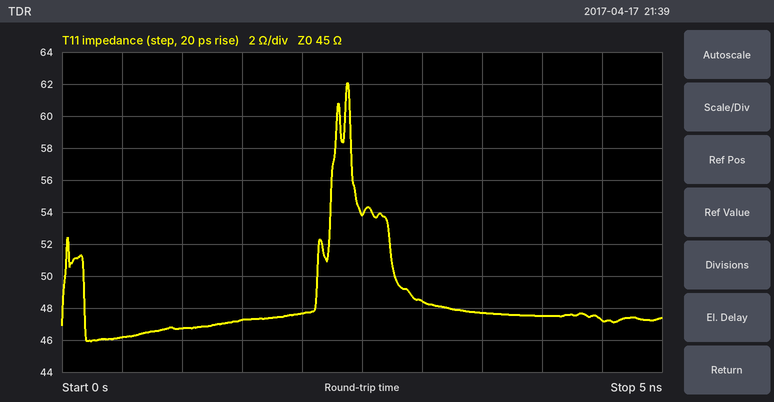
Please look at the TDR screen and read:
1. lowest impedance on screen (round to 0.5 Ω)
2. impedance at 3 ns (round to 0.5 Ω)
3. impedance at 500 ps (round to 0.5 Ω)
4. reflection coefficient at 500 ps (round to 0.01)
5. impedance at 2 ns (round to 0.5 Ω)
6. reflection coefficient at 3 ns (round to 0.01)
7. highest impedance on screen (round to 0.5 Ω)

46.0 Ω
48.5 Ω
46.0 Ω
+0.01
47.5 Ω
+0.04
62.0 Ω
